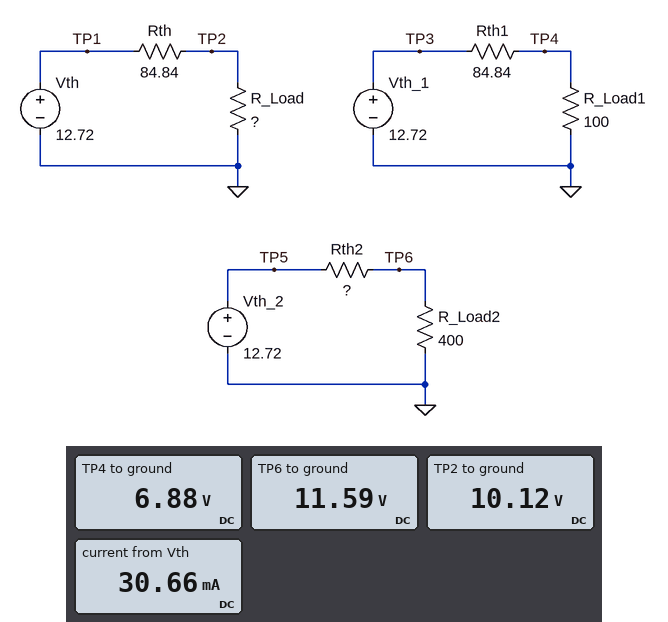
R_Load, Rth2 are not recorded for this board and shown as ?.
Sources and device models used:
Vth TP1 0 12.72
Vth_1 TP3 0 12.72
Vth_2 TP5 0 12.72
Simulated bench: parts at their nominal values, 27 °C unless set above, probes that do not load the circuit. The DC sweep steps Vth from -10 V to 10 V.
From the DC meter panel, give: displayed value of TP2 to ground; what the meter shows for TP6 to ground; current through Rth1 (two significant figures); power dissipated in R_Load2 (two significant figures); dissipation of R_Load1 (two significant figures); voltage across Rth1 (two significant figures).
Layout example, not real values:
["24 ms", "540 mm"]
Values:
["10.12 V", "11.59 V", "69 mA", "340 mW", "470 mW", "5.8 V"]
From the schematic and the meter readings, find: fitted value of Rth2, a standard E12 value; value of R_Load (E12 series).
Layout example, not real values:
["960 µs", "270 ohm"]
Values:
["39 Ω", "330 Ω"]
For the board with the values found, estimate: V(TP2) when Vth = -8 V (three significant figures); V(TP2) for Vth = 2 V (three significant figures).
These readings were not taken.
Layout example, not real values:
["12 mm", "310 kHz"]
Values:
["-6.36 V", "1.59 V"]
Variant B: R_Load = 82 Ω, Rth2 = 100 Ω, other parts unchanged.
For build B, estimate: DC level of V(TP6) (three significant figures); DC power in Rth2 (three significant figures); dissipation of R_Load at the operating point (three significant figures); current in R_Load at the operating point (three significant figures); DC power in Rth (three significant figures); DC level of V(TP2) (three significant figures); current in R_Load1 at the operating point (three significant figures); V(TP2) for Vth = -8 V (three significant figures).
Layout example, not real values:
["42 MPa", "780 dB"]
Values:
["10.2 V", "64.7 mW", "477 mW", "76.2 mA", "493 mW", "6.25 V", "68.8 mA", "-3.93 V"]
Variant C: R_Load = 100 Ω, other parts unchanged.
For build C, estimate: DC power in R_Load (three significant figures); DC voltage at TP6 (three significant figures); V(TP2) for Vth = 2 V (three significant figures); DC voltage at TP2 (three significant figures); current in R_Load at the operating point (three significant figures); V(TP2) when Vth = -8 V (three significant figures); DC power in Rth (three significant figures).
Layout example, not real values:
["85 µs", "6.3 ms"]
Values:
["474 mW", "11.6 V", "1.08 V", "6.88 V", "68.8 mA", "-4.33 V", "402 mW"]
